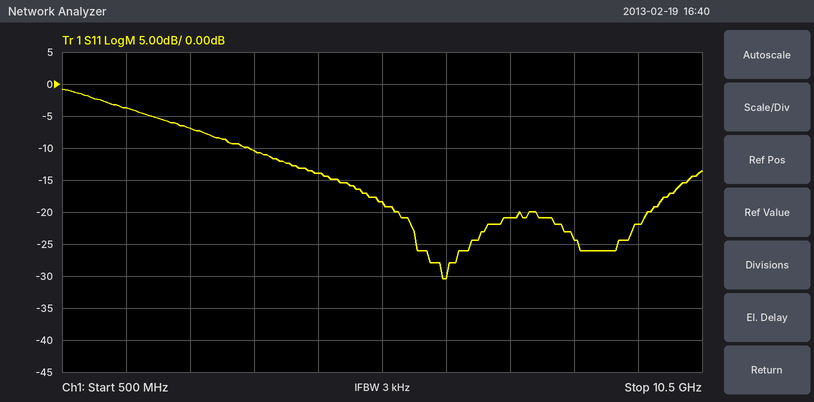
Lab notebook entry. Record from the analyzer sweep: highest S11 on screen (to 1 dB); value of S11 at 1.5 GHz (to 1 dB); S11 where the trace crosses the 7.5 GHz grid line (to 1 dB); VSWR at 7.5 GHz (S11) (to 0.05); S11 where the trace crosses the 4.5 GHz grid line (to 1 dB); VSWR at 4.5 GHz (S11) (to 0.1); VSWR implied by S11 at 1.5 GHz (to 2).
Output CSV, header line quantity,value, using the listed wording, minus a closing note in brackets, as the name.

quantity,value
highest S11 on screen,-1 dB
value of S11 at 1.5 GHz,-4 dB
S11 where the trace crosses the 7.5 GHz grid line,-21 dB
VSWR at 7.5 GHz (S11),1.20
S11 where the trace crosses the 4.5 GHz grid line,-14 dB
VSWR at 4.5 GHz (S11),1.5
VSWR implied by S11 at 1.5 GHz,4
